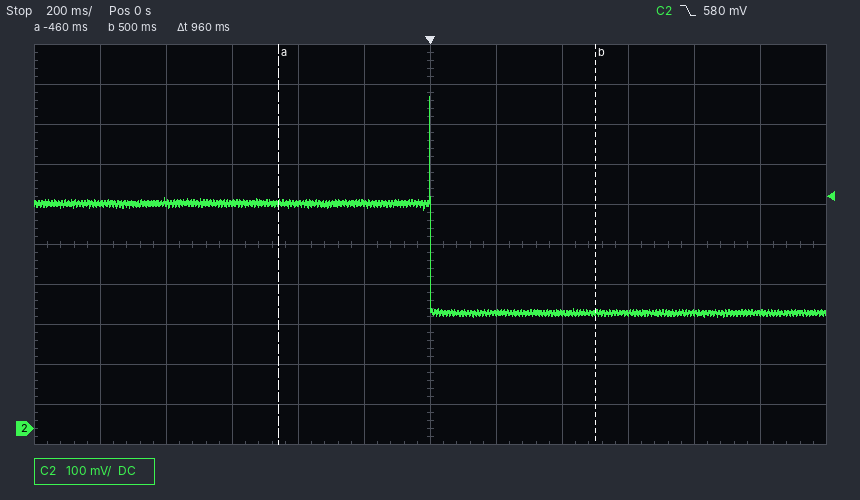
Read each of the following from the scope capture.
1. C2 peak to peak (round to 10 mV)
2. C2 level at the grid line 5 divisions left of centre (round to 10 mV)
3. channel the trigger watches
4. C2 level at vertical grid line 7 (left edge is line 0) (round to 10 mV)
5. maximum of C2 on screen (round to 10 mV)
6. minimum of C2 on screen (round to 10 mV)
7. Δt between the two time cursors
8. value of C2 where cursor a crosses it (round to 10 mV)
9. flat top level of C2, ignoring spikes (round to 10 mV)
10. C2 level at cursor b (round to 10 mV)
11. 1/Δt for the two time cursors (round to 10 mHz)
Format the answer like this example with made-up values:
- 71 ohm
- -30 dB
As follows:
- 550 mV
- 560 mV
- C2
- 290 mV
- 830 mV
- 280 mV
- 960 ms
- 560 mV
- 560 mV
- 290 mV
- 1.04 Hz
